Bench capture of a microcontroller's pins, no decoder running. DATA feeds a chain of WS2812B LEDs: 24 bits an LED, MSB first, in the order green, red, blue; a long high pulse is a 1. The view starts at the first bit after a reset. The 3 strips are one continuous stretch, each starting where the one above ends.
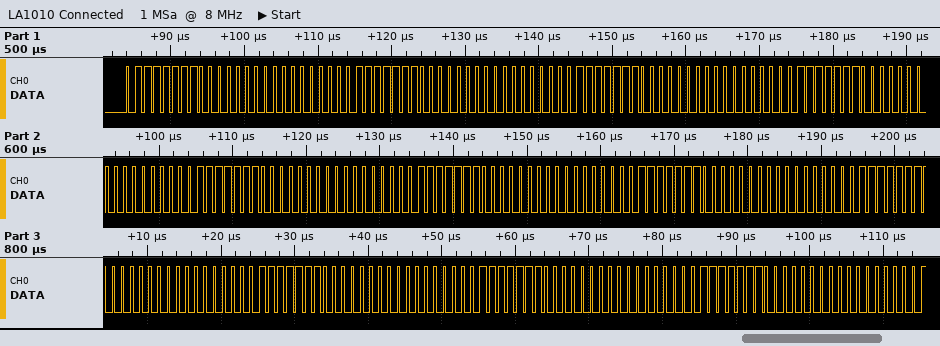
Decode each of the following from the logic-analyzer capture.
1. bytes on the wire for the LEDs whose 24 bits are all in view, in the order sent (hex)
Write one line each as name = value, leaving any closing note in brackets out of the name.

bytes on the wire for the LEDs whose 24 bits are all in view, in the order sent = 7F 00 00 7F 00 00 7F 00 00 7F 00 00 7F 00 00 7F 00 00 7F 00 00 7F 00 00 7F 00 00 7F 00 00 7F 00 00
